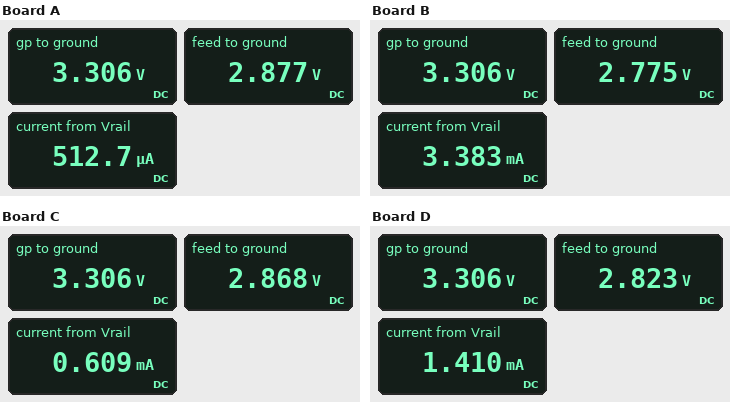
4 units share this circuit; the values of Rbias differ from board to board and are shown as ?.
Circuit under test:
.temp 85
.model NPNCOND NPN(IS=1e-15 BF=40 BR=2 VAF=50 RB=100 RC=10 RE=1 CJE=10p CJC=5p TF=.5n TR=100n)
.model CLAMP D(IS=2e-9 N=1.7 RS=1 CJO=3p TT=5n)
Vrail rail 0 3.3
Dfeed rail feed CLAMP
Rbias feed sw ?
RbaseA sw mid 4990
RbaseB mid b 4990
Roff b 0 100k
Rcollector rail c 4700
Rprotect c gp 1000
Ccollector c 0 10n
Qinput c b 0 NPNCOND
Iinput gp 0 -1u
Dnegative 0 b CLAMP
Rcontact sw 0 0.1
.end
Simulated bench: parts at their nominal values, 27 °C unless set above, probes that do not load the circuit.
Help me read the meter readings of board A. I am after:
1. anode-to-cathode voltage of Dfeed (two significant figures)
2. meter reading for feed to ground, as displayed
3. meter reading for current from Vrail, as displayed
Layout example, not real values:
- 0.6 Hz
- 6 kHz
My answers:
- 420 mV
- 2.877 V
- 512.7 µA
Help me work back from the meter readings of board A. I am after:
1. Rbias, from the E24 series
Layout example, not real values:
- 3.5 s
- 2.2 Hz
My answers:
- 5.6 kΩ
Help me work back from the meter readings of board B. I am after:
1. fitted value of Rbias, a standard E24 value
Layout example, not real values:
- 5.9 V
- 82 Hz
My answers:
- 820 Ω
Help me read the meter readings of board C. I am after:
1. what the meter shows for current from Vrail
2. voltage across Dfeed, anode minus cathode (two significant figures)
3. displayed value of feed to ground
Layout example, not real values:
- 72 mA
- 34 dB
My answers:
- 0.609 mA
- 430 mV
- 2.868 V
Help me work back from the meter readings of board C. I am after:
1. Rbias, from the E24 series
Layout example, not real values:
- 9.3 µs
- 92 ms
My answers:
- 4.7 kΩ
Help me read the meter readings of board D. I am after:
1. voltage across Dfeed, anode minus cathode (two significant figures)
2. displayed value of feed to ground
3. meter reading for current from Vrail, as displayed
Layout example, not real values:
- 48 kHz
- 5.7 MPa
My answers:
- 480 mV
- 2.823 V
- 1.410 mA
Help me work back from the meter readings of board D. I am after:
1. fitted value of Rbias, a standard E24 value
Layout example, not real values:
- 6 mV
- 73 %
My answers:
- 2 kΩ
